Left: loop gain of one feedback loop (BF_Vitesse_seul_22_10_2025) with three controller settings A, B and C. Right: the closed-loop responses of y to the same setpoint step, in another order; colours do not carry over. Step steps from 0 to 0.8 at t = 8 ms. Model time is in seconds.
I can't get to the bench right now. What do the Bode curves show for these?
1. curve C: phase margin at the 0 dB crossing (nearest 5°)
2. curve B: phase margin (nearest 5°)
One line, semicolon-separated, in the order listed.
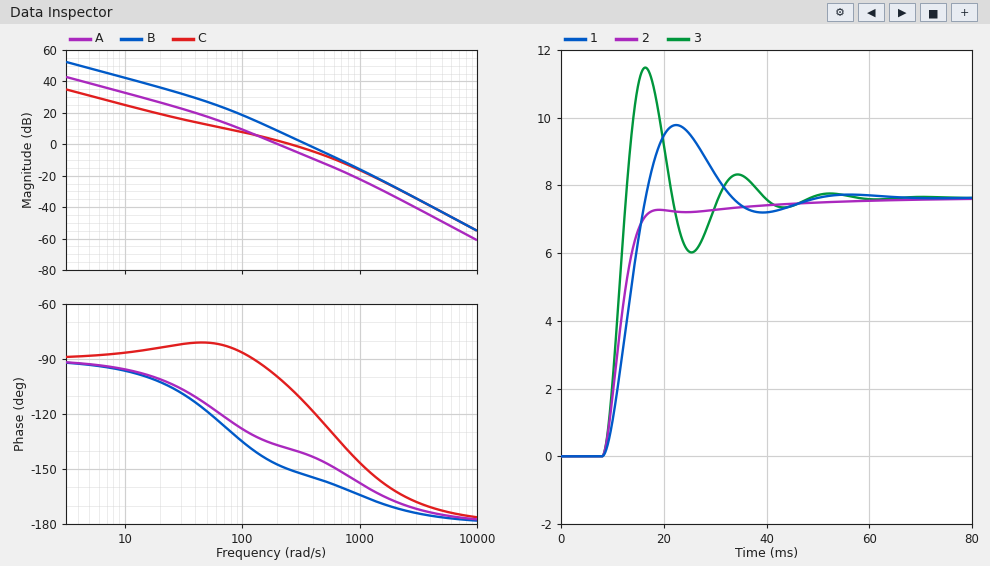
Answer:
75°; 25°
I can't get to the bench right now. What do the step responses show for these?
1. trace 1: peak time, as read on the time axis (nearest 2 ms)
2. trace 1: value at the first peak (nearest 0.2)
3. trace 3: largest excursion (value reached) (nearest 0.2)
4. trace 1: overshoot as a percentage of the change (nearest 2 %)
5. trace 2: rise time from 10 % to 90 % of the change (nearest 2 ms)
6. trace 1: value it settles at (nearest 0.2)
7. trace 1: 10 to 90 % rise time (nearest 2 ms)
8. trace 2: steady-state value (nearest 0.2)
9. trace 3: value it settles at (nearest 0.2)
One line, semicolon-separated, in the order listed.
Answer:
22 ms; 9.8; 11.4; 28 %; 6 ms; 7.6; 6 ms; 7.6; 7.6
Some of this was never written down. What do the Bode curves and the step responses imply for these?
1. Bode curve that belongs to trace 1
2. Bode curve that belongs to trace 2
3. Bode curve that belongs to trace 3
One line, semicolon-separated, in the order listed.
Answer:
A; C; B
